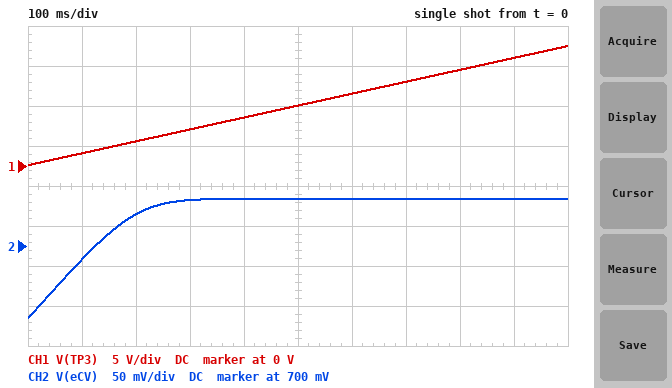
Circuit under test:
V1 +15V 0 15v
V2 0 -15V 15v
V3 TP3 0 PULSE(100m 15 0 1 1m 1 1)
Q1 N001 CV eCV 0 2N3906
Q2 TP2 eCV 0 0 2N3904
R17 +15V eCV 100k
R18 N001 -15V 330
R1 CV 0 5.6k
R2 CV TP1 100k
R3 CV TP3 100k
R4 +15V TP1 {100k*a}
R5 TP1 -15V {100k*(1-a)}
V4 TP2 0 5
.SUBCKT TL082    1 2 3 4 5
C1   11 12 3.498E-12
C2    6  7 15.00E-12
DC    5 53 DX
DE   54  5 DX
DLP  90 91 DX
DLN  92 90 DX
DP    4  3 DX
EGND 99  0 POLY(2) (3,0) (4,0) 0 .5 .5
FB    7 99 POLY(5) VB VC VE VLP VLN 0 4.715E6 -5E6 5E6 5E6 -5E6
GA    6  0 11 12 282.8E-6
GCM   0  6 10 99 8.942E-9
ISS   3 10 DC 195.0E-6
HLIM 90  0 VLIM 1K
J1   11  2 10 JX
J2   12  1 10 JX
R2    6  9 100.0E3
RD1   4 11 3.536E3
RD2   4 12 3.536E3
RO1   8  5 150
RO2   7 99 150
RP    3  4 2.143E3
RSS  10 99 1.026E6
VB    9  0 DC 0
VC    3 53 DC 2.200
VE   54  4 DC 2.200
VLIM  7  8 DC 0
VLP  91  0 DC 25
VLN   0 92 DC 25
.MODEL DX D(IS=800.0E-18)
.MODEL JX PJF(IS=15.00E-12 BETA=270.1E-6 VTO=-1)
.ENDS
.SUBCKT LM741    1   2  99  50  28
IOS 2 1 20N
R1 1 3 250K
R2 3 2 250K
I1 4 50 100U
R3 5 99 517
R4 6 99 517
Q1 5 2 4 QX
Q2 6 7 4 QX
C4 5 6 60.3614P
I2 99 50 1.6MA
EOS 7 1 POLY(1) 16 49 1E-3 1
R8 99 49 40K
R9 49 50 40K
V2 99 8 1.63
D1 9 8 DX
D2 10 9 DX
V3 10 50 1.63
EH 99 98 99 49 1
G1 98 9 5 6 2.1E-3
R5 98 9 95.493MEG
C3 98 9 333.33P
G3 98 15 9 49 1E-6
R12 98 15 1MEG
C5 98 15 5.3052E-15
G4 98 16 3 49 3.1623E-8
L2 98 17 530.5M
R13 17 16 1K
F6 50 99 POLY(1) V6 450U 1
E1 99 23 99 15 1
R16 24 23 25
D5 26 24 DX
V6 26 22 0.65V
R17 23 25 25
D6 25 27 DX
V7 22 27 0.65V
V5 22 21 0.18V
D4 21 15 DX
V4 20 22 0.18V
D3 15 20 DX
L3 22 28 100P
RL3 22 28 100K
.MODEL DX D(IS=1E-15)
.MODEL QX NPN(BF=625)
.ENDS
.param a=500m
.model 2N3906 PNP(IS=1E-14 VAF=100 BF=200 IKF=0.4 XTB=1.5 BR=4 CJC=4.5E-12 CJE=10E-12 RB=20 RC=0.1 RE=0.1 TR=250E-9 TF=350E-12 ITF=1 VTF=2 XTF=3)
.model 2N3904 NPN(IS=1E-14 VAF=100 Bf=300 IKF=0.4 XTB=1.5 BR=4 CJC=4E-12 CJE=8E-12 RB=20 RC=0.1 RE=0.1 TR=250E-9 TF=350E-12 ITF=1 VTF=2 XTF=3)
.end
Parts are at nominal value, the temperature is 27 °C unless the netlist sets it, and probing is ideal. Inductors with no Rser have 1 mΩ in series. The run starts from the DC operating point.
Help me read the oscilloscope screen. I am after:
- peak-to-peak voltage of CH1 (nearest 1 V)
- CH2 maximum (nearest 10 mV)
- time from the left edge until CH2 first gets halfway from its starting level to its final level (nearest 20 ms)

15 V
760 mV
100 ms
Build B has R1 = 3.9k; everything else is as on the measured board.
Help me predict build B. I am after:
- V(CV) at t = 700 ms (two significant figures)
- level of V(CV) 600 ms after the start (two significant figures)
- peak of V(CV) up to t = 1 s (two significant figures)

380 mV
330 mV
550 mV
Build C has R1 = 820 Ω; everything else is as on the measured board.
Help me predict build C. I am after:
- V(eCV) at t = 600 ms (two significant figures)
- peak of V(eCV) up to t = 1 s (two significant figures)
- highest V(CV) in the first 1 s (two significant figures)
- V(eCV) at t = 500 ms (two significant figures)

670 mV
720 mV
120 mV
660 mV
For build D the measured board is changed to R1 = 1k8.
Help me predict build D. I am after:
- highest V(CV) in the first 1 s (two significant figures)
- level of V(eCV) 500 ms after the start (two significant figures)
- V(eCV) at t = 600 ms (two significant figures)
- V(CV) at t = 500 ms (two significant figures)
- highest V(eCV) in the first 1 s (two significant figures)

260 mV
720 mV
740 mV
130 mV
760 mV
